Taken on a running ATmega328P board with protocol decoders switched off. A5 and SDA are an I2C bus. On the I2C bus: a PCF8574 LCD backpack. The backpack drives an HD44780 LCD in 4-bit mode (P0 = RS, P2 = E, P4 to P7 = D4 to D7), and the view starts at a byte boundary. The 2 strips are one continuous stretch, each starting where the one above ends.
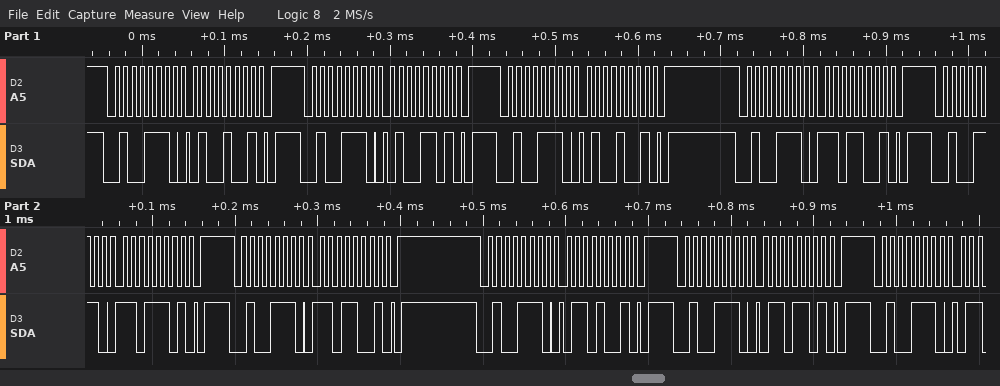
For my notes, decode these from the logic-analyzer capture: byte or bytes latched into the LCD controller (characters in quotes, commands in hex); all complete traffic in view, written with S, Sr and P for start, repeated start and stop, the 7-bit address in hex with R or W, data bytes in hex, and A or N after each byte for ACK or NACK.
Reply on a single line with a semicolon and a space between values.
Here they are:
'M'; S 27W A 49 A P S 27W A 4D A P S 27W A 49 A P S 27W A D9 A P S 27W A DD A P S 27W A D9 A P S 27W A 69 A P S 27W A 6D A P S 27W A
